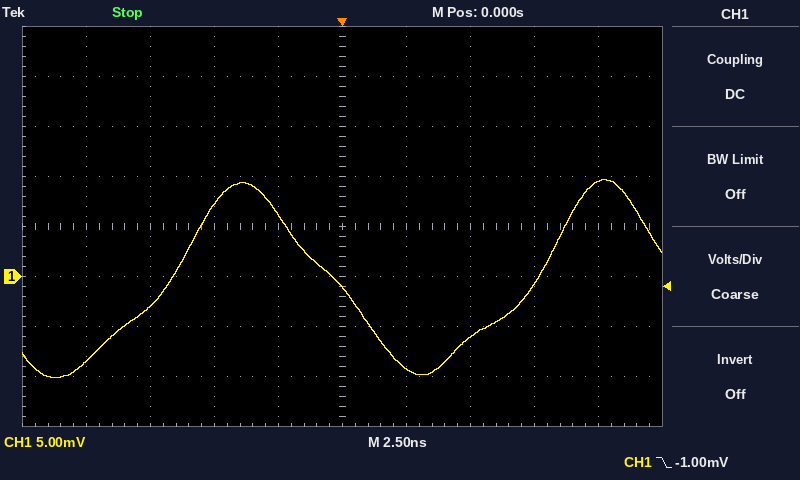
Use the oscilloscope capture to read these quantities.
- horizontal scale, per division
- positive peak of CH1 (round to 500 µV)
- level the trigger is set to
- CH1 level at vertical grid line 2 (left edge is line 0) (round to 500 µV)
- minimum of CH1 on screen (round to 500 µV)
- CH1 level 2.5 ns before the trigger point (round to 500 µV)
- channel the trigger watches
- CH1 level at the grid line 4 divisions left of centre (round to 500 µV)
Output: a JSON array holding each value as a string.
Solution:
["2.5 ns", "9.5 mV", "-1.00 mV", "-3.0 mV", "-10.0 mV", "6.0 mV", "CH1", "-8.5 mV"]
